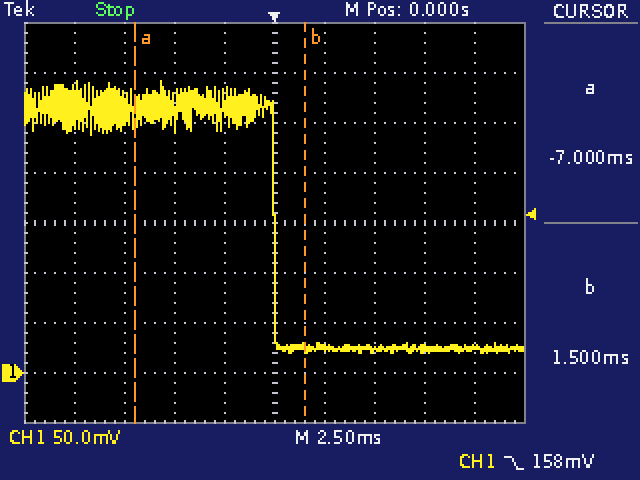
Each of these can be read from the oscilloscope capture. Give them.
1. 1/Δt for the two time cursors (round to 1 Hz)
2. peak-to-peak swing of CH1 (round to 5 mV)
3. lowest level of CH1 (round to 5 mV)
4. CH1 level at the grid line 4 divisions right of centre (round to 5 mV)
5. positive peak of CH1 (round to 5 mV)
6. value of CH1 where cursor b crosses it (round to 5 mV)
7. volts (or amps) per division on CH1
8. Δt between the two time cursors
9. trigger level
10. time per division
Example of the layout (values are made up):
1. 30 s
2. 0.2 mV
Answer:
1. 118 Hz
2. 270 mV
3. 20 mV
4. 25 mV
5. 290 mV
6. 25 mV
7. 50 mV
8. 8.50 ms
9. 158 mV
10. 2.5 ms
